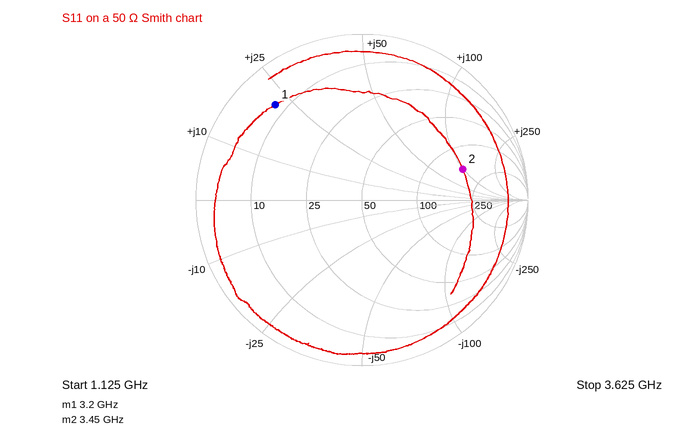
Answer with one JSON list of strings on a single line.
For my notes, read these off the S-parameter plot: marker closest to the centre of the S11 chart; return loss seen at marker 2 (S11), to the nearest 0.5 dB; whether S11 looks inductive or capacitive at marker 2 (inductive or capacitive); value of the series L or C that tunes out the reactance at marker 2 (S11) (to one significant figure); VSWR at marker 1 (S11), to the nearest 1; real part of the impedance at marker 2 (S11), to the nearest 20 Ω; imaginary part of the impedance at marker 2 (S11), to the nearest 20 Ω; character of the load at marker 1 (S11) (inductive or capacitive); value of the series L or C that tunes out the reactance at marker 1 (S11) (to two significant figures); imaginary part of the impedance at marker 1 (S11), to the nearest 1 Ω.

["marker 2", "4.0 dB", "inductive", "500 fF", "8", "160 Ω", "+100 Ω", "inductive", "2.3 pF", "+22 Ω"]
